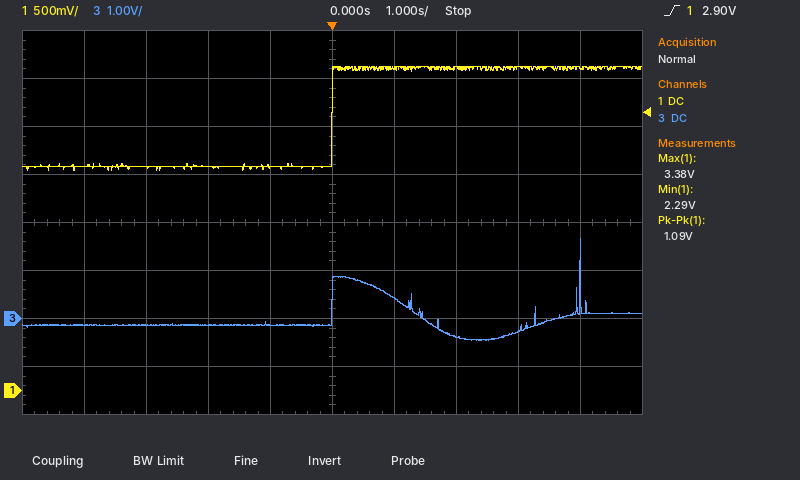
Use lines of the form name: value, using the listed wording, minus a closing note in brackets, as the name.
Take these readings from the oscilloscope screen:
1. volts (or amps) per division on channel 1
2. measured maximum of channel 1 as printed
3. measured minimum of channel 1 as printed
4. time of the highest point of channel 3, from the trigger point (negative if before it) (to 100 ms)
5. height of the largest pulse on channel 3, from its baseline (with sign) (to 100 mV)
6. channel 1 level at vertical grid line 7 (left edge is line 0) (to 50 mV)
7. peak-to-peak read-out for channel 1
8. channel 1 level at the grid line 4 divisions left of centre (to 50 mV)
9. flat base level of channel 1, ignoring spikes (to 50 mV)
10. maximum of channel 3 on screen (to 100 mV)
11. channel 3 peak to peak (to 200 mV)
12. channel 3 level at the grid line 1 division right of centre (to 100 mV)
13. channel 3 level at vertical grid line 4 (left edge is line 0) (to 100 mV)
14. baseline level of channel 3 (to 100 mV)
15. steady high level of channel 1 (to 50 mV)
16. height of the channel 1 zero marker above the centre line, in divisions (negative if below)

volts (or amps) per division on channel 1: 500 mV
measured maximum of channel 1 as printed: 3.38 V
measured minimum of channel 1 as printed: 2.29 V
time of the highest point of channel 3, from the trigger point (negative if before it): +4.0 s
height of the largest pulse on channel 3, from its baseline (with sign): +1.8 V
channel 1 level at vertical grid line 7 (left edge is line 0): 3.35 V
peak-to-peak read-out for channel 1: 1.09 V
channel 1 level at the grid line 4 divisions left of centre: 2.35 V
flat base level of channel 1, ignoring spikes: 2.35 V
maximum of channel 3 on screen: 1.7 V
channel 3 peak to peak: 2.2 V
channel 3 level at the grid line 1 division right of centre: 400 mV
channel 3 level at vertical grid line 4 (left edge is line 0): -100 mV
baseline level of channel 3: -100 mV
steady high level of channel 1: 3.35 V
height of the channel 1 zero marker above the centre line, in divisions: -3.5 div
